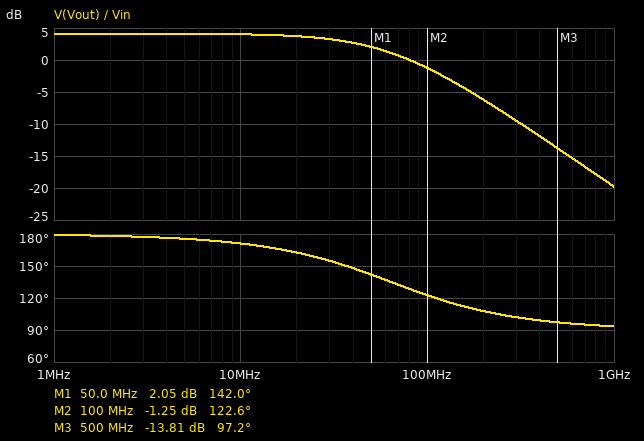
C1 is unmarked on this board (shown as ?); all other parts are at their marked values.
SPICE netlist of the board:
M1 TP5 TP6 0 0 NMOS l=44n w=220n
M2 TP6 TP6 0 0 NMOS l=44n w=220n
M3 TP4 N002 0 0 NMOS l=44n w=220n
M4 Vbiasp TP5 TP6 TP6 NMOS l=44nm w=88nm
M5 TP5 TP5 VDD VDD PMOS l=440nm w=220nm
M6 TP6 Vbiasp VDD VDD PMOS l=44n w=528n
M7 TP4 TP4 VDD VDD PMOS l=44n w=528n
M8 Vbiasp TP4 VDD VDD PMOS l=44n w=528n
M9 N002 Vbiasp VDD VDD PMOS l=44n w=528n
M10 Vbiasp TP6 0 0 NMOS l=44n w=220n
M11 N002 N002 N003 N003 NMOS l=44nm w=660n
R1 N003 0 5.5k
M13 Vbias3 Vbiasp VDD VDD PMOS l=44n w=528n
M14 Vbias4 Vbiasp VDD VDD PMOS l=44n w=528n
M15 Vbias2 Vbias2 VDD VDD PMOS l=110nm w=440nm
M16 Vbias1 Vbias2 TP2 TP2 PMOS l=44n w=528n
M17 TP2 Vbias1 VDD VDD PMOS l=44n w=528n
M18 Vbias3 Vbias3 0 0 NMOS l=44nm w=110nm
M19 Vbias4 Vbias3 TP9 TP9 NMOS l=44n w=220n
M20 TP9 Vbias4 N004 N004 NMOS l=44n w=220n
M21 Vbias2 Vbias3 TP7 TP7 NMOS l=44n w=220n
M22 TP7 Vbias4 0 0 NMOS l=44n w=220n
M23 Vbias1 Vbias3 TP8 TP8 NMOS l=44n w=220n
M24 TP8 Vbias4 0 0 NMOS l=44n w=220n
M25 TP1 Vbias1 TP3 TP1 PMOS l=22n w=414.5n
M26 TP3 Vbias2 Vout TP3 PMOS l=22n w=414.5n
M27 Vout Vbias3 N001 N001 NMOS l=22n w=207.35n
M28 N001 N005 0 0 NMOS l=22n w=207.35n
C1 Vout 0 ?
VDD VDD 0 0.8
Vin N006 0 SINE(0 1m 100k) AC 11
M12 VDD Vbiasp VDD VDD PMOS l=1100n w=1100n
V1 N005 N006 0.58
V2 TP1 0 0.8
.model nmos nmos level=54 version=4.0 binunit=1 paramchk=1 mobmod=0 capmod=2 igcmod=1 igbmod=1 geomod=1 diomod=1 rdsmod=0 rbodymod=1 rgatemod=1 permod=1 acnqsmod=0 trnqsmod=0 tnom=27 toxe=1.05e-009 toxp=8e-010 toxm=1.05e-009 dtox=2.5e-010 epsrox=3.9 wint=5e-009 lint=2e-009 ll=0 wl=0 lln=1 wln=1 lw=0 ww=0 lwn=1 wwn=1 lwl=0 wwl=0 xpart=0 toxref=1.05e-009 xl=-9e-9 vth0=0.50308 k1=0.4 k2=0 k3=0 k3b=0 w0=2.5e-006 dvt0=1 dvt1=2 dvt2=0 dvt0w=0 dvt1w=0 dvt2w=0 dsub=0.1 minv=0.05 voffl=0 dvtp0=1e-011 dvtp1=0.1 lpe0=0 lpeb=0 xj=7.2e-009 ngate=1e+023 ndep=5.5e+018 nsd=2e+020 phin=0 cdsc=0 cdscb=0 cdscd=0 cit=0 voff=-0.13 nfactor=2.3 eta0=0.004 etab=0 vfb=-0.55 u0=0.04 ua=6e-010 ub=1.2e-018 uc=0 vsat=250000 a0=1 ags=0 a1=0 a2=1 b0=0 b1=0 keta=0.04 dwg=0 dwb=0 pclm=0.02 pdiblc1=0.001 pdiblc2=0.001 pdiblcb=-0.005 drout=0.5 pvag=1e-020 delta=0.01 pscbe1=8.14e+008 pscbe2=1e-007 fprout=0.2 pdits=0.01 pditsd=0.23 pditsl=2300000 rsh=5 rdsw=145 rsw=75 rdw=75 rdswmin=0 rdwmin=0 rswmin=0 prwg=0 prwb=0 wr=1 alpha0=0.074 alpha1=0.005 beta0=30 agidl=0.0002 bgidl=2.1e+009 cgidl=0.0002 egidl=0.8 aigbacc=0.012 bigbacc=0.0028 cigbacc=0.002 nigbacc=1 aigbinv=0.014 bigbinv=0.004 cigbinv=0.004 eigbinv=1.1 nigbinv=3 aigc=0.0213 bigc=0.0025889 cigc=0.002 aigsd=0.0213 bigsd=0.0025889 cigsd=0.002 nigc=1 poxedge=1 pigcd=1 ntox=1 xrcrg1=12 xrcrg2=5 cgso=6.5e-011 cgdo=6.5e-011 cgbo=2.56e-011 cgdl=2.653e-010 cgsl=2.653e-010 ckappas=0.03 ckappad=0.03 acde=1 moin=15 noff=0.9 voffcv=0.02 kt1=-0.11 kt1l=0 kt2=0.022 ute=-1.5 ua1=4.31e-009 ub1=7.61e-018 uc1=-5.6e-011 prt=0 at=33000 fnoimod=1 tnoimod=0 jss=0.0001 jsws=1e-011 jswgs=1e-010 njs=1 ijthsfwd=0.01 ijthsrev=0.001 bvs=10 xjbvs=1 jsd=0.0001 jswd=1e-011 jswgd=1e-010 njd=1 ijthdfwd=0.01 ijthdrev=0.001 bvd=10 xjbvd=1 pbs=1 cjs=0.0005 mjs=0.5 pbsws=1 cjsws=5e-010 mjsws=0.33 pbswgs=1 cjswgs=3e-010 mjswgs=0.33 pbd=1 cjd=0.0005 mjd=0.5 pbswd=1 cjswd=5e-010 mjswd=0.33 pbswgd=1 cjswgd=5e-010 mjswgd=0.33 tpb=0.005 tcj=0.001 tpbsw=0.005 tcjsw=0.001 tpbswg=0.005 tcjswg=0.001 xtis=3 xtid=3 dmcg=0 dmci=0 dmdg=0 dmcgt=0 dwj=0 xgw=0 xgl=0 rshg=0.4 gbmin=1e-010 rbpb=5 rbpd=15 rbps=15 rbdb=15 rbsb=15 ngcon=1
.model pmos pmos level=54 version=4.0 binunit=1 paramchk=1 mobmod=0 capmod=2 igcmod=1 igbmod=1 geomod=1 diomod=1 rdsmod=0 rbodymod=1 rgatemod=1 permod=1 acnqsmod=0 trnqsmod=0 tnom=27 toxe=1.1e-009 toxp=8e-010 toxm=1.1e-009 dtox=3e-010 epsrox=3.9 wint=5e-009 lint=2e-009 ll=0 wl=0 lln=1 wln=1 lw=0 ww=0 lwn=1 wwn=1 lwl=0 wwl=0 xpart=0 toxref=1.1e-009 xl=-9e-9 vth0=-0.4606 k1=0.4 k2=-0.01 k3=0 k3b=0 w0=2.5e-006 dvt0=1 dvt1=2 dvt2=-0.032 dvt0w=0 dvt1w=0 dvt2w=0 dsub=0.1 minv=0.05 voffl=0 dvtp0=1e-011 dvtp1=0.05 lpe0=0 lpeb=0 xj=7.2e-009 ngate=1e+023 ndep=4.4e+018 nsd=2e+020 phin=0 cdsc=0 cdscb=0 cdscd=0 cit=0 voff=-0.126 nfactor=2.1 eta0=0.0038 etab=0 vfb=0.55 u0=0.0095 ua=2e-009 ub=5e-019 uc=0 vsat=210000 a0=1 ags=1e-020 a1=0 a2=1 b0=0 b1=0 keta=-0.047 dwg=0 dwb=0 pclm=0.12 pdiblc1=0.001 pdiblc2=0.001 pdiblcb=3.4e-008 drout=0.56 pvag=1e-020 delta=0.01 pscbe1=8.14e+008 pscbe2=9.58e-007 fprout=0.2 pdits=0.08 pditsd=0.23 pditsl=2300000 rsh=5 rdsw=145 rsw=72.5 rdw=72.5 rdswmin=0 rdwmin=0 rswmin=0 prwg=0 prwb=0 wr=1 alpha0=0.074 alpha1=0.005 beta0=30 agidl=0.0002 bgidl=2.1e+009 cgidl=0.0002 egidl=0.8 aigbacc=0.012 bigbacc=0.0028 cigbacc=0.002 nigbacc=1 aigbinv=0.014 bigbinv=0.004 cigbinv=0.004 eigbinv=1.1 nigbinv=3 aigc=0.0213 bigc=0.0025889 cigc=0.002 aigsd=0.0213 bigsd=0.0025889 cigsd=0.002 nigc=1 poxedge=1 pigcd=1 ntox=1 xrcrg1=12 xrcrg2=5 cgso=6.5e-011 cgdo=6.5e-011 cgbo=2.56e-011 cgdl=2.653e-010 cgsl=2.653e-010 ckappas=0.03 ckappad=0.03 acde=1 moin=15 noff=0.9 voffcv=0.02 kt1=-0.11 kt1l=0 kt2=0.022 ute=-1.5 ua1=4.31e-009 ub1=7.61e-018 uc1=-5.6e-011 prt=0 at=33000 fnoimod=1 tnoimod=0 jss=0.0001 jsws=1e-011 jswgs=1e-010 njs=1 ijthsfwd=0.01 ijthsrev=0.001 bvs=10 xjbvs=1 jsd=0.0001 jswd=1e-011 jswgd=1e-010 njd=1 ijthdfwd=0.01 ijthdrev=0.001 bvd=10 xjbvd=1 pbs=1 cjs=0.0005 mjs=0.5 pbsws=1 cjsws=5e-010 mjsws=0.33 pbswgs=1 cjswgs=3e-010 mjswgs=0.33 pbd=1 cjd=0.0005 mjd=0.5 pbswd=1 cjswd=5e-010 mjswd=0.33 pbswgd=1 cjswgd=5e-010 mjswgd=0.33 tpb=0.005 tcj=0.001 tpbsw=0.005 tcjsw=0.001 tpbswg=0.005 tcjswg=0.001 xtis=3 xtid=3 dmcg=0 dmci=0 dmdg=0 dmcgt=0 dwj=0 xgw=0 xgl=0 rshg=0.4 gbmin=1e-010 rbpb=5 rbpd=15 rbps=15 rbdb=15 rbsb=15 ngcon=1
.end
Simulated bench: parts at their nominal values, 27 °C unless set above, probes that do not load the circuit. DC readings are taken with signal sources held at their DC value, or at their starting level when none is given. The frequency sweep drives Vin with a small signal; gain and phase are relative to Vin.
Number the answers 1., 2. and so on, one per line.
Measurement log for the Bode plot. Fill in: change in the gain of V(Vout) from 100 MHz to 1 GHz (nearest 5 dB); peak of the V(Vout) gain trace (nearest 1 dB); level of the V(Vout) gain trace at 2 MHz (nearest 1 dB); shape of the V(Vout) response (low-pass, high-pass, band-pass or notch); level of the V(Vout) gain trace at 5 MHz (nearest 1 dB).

1. -20 dB
2. 4 dB
3. 4 dB
4. low-pass
5. 4 dB
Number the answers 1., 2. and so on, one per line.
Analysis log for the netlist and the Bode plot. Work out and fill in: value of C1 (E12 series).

1. 390 fF
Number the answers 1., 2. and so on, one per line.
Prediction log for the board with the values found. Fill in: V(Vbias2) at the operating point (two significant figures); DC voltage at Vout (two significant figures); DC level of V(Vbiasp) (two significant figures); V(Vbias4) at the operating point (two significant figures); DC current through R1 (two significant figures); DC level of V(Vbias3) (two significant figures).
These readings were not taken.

1. 93 mV
2. 570 mV
3. 230 mV
4. 800 mV
5. 12 µA
6. 610 mV
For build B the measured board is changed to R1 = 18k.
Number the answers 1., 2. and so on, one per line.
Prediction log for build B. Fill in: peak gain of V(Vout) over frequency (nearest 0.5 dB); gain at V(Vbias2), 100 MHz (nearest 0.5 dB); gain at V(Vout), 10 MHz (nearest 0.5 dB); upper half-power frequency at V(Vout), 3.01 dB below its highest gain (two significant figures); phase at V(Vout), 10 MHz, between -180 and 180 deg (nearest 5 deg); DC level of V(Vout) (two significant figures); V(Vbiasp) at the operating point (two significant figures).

1. 2.0 dB
2. -67.0 dB
3. 1.5 dB
4. 29 MHz
5. 160 deg
6. 420 mV
7. 320 mV
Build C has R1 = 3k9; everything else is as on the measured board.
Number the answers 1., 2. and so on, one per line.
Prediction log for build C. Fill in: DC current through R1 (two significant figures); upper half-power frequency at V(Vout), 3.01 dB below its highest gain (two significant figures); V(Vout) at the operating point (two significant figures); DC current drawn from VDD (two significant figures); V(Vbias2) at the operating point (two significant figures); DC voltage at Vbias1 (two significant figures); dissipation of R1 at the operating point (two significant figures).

1. 19 µA
2. 78 MHz
3. 580 mV
4. 120 µA
5. 79 mV
6. 160 mV
7. 1.4 µW
